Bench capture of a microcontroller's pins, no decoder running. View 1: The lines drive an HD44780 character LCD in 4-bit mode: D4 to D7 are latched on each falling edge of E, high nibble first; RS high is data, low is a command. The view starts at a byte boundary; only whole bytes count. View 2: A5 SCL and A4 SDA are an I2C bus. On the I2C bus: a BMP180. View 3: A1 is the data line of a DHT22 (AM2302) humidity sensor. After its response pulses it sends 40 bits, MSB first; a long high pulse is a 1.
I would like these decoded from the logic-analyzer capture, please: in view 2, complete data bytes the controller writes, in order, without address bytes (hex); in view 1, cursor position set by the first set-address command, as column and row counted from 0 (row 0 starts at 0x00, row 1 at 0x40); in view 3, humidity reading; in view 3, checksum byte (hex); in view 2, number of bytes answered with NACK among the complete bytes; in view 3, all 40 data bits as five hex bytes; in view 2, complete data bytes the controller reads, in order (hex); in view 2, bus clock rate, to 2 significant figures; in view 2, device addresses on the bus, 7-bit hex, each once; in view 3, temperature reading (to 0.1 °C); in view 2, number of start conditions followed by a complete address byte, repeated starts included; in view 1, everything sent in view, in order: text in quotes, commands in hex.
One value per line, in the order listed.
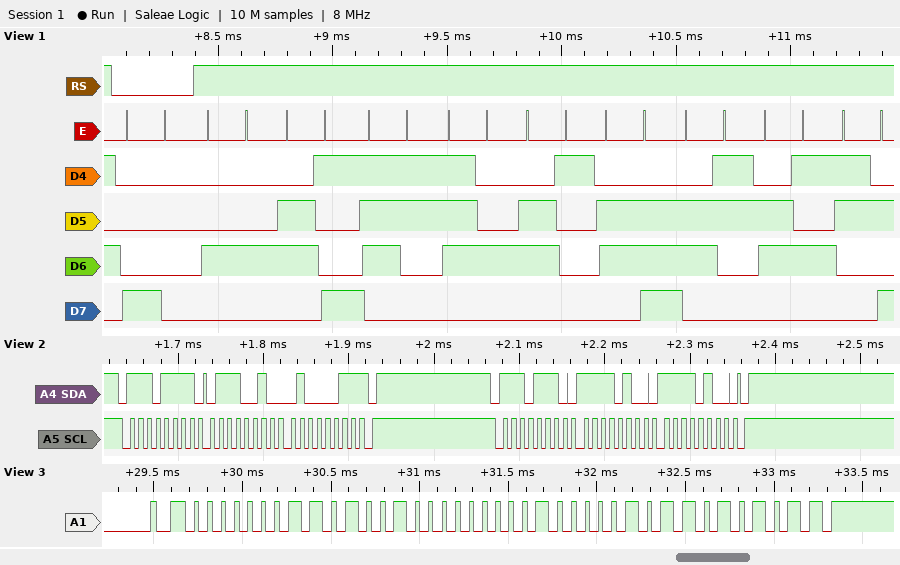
F4 F4
column 0, row 0
42.0 %
0xAB
1
01 A4 01 05 AB
72 43
100 kHz
0x77
26.1 °C
2
0x80 "Distance:"
